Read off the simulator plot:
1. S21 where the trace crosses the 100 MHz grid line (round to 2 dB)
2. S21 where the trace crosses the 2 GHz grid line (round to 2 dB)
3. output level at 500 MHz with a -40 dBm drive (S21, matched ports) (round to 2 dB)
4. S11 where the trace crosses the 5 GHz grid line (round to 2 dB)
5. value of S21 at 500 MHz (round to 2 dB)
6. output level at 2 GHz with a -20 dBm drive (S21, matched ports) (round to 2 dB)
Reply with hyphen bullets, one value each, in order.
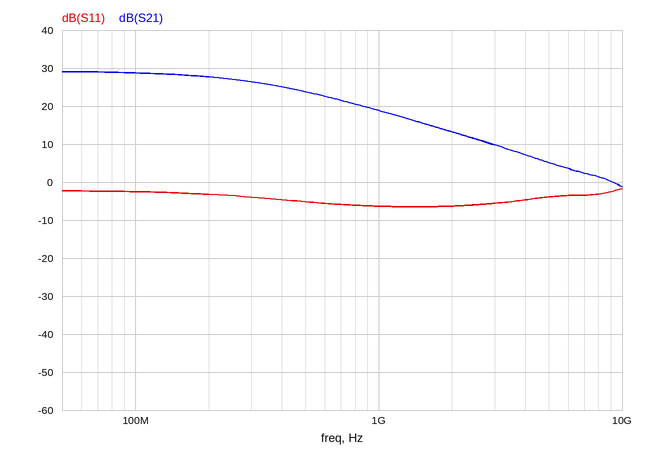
- 28 dB
- 14 dB
- -16 dBm
- -4 dB
- 24 dB
- -6 dBm
